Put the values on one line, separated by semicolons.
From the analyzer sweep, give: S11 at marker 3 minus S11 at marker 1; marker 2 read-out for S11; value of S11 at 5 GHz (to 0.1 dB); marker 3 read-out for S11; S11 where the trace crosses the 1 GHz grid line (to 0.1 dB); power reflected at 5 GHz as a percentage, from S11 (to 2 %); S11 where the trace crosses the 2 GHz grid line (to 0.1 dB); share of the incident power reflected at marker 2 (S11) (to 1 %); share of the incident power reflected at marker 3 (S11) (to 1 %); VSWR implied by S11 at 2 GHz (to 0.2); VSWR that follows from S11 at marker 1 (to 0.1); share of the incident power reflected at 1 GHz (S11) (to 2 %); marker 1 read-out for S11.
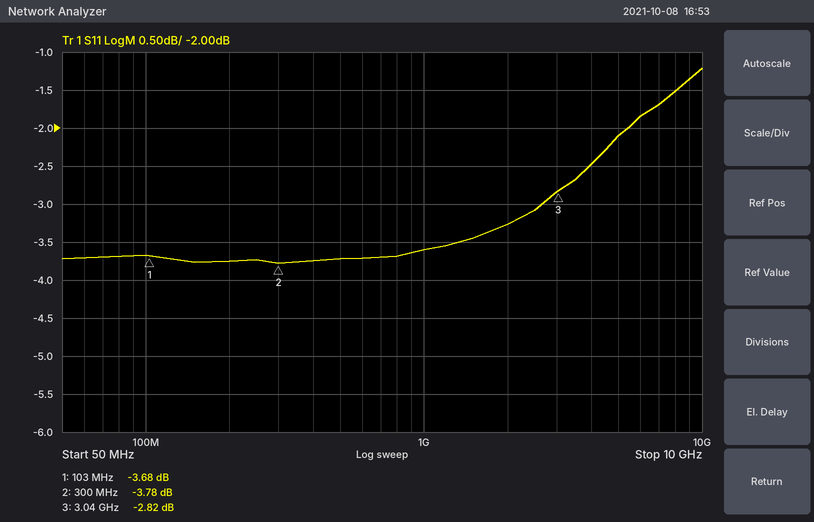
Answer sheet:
0.86 dB; -3.78 dB; -2.1 dB; -2.82 dB; -3.6 dB; 62 %; -3.3 dB; 42 %; 52 %; 5.4; 4.8; 44 %; -3.68 dB
